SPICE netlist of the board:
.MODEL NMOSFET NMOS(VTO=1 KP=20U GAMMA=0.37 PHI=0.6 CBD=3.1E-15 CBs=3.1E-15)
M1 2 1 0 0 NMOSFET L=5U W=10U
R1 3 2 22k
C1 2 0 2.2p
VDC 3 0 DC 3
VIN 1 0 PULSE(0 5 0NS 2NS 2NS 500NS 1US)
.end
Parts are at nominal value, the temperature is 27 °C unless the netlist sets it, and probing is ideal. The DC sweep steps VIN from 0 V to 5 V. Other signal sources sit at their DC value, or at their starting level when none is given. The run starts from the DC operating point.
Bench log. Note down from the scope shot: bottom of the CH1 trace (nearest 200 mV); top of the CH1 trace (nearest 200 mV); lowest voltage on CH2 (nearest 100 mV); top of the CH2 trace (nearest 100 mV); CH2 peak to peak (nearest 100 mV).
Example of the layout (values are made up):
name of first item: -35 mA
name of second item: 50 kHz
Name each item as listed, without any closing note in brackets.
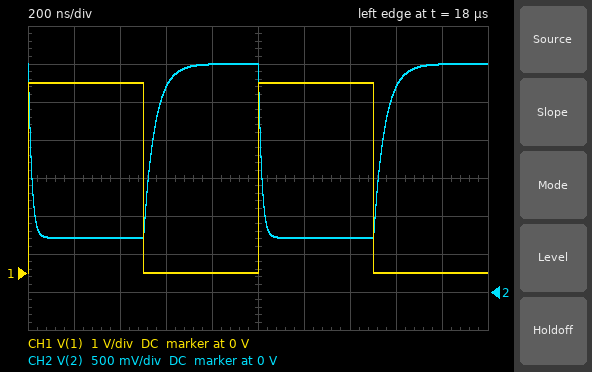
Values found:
bottom of the CH1 trace: 0 V
top of the CH1 trace: 5.0 V
lowest voltage on CH2: 700 mV
top of the CH2 trace: 3.0 V
CH2 peak to peak: 2.3 V
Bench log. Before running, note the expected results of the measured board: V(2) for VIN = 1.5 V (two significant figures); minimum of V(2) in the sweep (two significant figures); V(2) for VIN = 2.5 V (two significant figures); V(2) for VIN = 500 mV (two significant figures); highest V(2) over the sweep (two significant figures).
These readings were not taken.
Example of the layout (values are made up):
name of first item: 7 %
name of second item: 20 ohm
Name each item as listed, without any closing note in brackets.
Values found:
V(2) for VIN = 1.5 V: 2.9 V
minimum of V(2) in the sweep: 710 mV
V(2) for VIN = 2.5 V: 2.0 V
V(2) for VIN = 500 mV: 3.0 V
highest V(2) over the sweep: 3.0 V
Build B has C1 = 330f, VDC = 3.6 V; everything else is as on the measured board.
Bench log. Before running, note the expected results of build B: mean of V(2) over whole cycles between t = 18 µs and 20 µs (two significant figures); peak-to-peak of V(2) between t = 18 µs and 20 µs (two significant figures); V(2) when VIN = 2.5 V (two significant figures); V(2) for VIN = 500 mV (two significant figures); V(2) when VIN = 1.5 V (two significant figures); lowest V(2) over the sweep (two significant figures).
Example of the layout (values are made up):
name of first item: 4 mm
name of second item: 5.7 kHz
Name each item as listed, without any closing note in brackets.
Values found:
mean of V(2) over whole cycles between t = 18 µs and 20 µs: 2.2 V
peak-to-peak of V(2) between t = 18 µs and 20 µs: 2.7 V
V(2) when VIN = 2.5 V: 2.6 V
V(2) for VIN = 500 mV: 3.6 V
V(2) when VIN = 1.5 V: 3.5 V
lowest V(2) over the sweep: 870 mV
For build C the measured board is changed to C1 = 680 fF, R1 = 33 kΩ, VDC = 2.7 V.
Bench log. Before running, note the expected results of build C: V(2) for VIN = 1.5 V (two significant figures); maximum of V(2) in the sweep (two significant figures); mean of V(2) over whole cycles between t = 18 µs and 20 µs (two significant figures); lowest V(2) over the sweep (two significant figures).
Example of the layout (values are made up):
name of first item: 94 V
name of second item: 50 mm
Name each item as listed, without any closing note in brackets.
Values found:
V(2) for VIN = 1.5 V: 2.5 V
maximum of V(2) in the sweep: 2.7 V
mean of V(2) over whole cycles between t = 18 µs and 20 µs: 1.5 V
lowest V(2) over the sweep: 450 mV
